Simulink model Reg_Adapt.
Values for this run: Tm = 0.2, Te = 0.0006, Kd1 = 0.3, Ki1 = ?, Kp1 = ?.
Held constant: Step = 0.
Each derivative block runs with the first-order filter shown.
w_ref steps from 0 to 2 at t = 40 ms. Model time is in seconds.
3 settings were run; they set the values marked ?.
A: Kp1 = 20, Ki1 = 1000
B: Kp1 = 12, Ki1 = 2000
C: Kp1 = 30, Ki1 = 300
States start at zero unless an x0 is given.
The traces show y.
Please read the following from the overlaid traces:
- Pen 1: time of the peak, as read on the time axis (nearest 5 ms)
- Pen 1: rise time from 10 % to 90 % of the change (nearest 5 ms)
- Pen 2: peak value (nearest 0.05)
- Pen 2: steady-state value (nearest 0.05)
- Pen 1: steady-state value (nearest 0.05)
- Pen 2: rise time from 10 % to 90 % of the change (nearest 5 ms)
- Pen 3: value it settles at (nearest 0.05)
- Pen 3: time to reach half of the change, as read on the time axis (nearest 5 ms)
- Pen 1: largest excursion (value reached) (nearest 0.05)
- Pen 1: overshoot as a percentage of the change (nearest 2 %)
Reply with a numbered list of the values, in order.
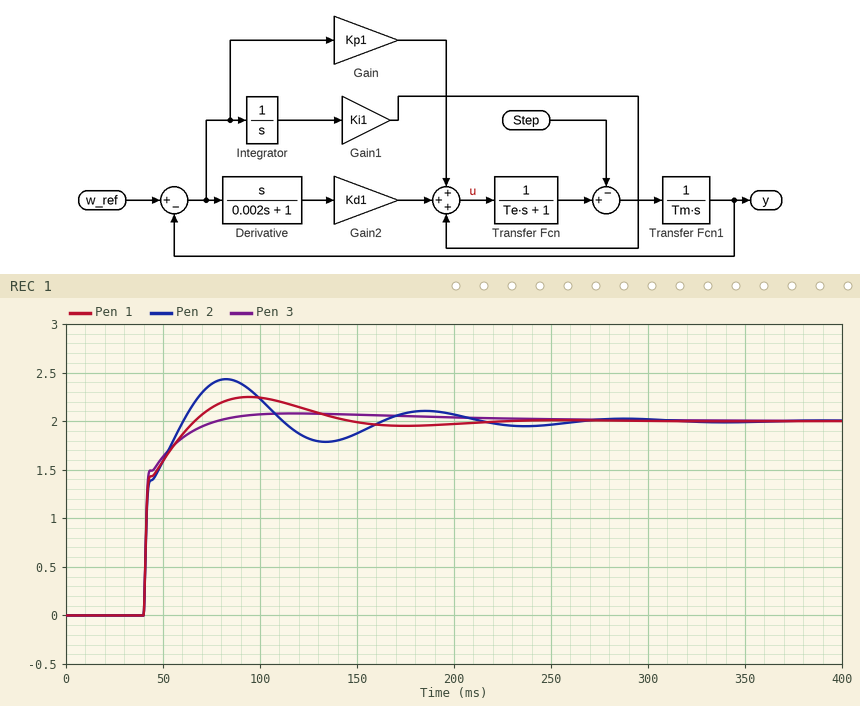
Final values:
1. 95 ms
2. 15 ms
3. 2.45
4. 2.00
5. 2.00
6. 15 ms
7. 2.00
8. 40 ms
9. 2.25
10. 12 %
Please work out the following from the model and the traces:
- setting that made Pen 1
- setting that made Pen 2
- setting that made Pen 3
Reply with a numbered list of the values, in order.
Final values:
1. A
2. B
3. C
